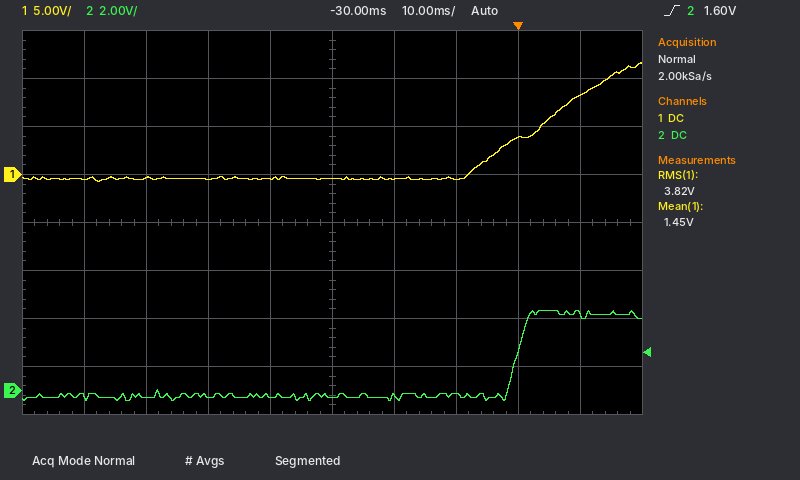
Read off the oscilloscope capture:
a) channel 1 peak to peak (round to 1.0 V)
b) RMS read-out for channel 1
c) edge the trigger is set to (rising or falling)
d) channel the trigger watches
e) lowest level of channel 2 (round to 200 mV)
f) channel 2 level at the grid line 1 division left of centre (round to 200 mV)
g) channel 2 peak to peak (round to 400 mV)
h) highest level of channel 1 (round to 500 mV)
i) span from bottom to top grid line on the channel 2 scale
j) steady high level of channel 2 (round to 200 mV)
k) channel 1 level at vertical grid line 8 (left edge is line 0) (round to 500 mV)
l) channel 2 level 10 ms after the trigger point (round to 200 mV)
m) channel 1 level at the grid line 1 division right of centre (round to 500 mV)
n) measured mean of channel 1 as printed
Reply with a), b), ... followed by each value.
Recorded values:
a) 12.0 V
b) 3.82 V
c) rising
d) channel 2
e) -400 mV
f) -200 mV
g) 3.6 V
h) 11.5 V
i) 16 V
j) 3.2 V
k) 4.0 V
l) 3.2 V
m) -500 mV
n) 1.45 V
